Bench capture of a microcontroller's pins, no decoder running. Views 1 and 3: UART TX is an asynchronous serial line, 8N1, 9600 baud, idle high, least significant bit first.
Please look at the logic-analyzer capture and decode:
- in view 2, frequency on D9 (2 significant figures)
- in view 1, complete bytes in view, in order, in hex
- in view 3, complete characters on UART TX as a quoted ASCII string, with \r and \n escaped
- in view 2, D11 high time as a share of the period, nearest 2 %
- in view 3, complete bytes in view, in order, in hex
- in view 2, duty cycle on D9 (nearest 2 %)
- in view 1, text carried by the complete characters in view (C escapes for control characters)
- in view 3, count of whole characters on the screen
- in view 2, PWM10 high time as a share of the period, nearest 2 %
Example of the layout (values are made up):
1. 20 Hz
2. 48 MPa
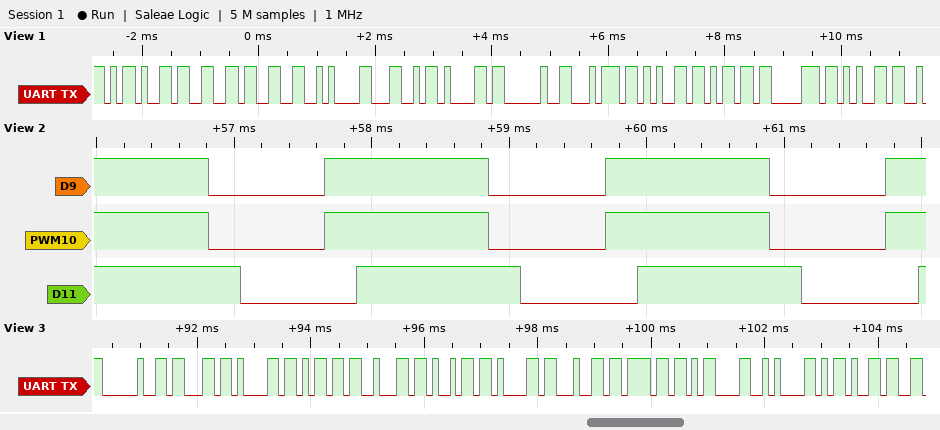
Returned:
1. 490 Hz
2. 0x2D 0x33 0x33 0x0A 0x4C 0x61 0x20 0x74 0x65 0x6D 0x70 0x65
3. " cambiado\r\n-"
4. 58 %
5. 20 63 61 6D 62 69 61 64 6F 0D 0A 2D
6. 58 %
7. "-33\nLa tempe"
8. 12
9. 58 %
